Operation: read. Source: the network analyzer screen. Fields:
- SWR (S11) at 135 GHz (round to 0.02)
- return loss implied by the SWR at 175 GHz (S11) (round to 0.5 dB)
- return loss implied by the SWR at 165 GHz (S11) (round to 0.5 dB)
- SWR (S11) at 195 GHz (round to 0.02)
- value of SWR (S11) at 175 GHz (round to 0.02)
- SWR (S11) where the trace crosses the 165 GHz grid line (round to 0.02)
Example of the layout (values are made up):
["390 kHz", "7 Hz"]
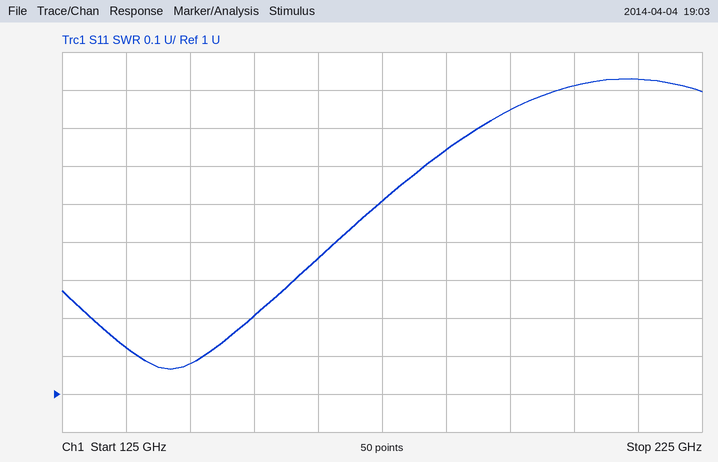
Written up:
["1.12", "14.0 dB", "16.5 dB", "1.74", "1.50", "1.36"]
